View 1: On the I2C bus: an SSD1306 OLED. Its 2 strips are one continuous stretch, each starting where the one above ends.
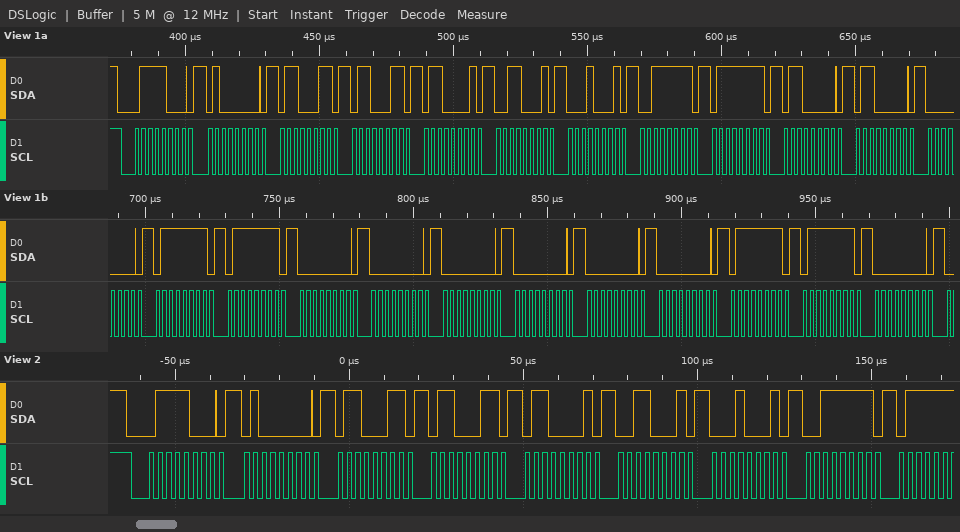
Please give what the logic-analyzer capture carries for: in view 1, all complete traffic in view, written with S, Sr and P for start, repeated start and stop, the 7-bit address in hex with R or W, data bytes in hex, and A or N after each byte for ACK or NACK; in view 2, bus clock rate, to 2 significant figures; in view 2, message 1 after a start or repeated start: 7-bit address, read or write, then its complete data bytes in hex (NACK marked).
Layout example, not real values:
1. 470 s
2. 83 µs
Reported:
1. S 3CW A 40 A 63 A 63 A 61 A 31 A 11 A 3F A 7F A 60 A 60 A 00 A 7F A 7F A 00 A 00 A 00 A 00 A 00 A 00 A 7F A 7F A 00 A
2. 400 kHz
3. 0x3C write: 40 63 63 61 31 11 3F
